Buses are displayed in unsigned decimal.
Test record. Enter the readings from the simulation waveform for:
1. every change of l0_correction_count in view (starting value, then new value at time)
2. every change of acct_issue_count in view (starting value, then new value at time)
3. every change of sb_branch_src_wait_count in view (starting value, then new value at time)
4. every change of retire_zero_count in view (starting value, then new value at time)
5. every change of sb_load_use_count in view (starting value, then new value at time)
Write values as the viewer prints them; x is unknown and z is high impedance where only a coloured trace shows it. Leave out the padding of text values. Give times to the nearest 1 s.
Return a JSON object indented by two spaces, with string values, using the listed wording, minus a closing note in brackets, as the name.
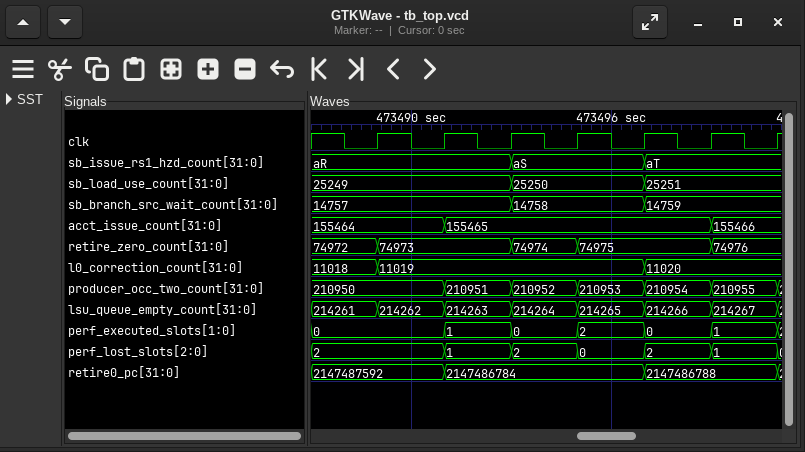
{
  "every change of l0_correction_count in view": "11018, 11019 at 473489 s, 11020 at 473497 s",
  "every change of acct_issue_count in view": "155464, 155465 at 473491 s, 155466 at 473499 s",
  "every change of sb_branch_src_wait_count in view": "14757, 14758 at 473493 s, 14759 at 473497 s",
  "every change of retire_zero_count in view": "74972, 74973 at 473489 s, 74974 at 473493 s, 74975 at 473495 s, 74976 at 473499 s",
  "every change of sb_load_use_count in view": "25249, 25250 at 473493 s, 25251 at 473497 s"
}
